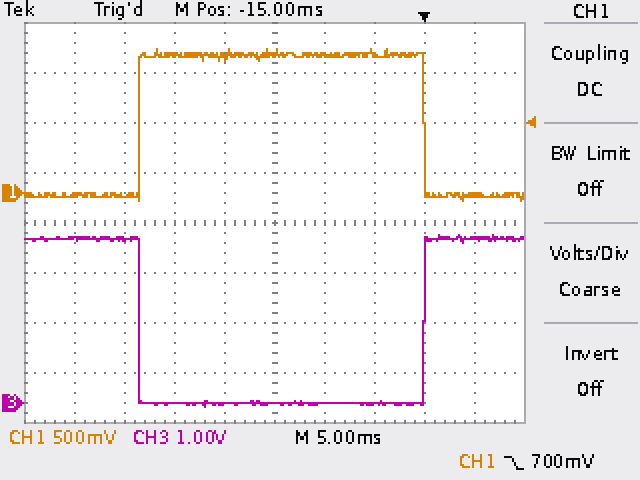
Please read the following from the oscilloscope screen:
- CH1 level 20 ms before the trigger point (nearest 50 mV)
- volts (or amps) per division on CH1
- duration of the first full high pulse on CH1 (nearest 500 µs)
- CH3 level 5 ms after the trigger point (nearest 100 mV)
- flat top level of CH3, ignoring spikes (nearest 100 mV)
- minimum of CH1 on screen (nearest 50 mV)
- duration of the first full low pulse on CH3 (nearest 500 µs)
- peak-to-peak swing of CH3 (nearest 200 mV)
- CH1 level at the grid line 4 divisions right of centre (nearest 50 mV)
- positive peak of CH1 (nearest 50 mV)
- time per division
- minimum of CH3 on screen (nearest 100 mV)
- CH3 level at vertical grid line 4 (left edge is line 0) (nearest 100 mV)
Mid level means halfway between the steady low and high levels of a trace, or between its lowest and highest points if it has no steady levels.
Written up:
1.35 V
500 mV
28.5 ms
3.3 V
3.3 V
-100 mV
28.5 ms
3.4 V
0 mV
1.45 V
5 ms
-100 mV
0.0 V
